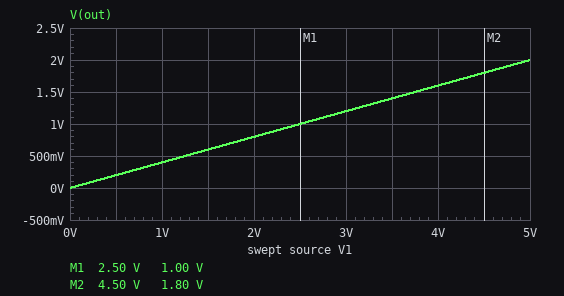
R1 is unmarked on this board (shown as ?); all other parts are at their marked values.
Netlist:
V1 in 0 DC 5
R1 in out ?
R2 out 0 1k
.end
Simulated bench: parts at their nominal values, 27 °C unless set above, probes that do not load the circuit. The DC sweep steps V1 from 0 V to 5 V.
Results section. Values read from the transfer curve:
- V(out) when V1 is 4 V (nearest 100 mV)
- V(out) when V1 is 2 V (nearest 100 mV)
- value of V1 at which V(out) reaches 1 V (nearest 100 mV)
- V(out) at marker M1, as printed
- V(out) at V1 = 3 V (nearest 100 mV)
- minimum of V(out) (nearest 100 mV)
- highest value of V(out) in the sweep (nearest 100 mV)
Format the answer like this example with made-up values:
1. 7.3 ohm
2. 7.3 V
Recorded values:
1. 1.6 V
2. 800 mV
3. 2.5 V
4. 1.00 V
5. 1.2 V
6. 0 V
7. 2.0 V
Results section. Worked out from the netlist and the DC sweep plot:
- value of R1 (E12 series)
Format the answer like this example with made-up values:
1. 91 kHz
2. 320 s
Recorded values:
1. 1.5 kΩ
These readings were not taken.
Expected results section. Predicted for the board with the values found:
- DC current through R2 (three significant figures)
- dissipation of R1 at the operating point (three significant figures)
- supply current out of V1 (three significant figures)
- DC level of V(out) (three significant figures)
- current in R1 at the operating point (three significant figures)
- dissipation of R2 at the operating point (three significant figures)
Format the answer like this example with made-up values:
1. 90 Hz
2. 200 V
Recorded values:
1. 2.00 mA
2. 6.00 mW
3. 2.00 mA
4. 2.00 V
5. 2.00 mA
6. 4.00 mW
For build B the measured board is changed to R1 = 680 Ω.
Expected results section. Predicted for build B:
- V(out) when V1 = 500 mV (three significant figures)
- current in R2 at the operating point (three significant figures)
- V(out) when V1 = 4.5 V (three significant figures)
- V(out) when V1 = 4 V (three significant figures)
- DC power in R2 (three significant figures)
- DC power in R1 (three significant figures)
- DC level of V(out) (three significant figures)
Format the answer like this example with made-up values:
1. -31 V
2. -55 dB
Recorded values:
1. 298 mV
2. 2.98 mA
3. 2.68 V
4. 2.38 V
5. 8.86 mW
6. 6.02 mW
7. 2.98 V
